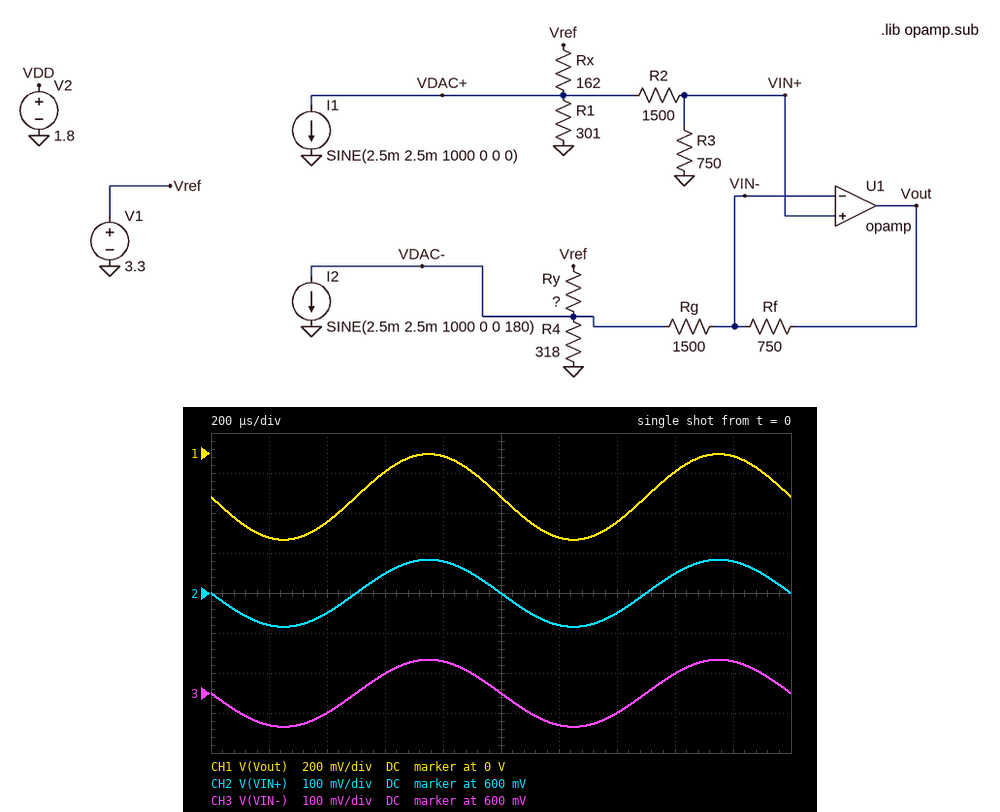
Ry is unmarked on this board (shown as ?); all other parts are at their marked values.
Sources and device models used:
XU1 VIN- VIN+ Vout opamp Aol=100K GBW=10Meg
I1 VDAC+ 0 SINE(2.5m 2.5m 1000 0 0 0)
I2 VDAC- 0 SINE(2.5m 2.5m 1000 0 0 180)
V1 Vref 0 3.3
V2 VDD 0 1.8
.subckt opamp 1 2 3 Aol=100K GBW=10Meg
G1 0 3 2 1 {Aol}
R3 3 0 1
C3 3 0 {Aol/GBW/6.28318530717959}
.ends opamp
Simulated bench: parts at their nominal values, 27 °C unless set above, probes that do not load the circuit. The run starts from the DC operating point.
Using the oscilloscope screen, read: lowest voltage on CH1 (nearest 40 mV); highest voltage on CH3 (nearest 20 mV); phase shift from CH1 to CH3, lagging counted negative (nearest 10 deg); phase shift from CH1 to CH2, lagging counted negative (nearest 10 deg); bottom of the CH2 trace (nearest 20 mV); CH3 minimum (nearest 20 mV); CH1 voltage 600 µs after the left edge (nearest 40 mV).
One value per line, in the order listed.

-440 mV
680 mV
0 deg
0 deg
520 mV
520 mV
-80 mV
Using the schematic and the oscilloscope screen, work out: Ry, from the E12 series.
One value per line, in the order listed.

100 Ω
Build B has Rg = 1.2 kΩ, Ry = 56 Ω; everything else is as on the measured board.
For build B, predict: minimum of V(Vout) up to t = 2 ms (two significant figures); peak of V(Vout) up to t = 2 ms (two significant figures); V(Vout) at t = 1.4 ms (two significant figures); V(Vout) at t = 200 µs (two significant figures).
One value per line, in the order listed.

-860 mV
-450 mV
-780 mV
-850 mV
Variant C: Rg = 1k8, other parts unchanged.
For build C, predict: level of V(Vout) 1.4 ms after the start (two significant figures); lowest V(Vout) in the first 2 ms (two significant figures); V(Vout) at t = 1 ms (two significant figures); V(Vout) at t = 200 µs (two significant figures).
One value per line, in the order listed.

-200 mV
-280 mV
-89 mV
-270 mV
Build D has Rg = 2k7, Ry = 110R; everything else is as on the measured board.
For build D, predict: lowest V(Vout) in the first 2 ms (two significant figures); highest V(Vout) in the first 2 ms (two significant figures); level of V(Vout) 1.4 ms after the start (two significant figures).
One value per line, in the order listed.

-6.6 mV
320 mV
60 mV
